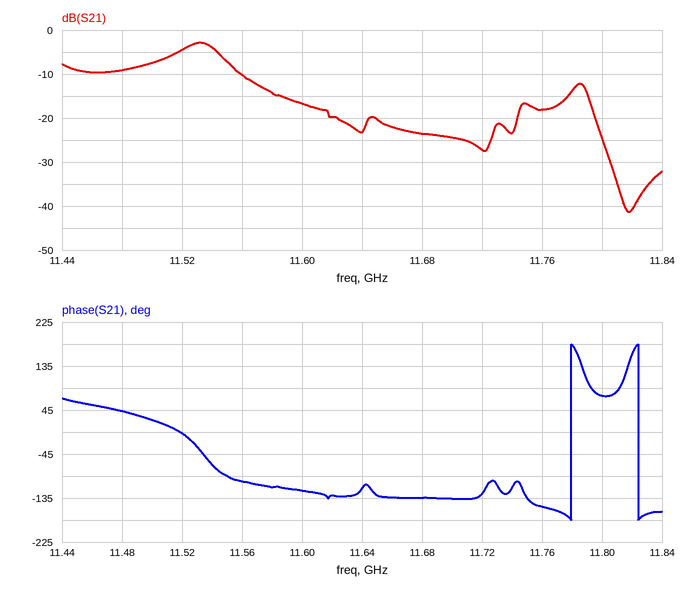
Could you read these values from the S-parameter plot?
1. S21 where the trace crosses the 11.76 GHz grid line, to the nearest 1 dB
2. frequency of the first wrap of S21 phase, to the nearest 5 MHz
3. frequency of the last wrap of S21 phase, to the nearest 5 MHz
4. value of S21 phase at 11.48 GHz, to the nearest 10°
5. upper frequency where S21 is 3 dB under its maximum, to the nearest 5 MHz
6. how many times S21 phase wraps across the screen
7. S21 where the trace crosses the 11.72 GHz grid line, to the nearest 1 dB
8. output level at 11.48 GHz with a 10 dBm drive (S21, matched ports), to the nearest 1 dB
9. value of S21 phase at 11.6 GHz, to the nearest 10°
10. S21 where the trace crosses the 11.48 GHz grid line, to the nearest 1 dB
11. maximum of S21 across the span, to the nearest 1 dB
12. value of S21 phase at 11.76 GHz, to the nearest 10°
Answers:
-18 dB
11.780 GHz
11.825 GHz
40°
11.545 GHz
2
-27 dB
1 dBm
-120°
-9 dB
-3 dB
-150°
